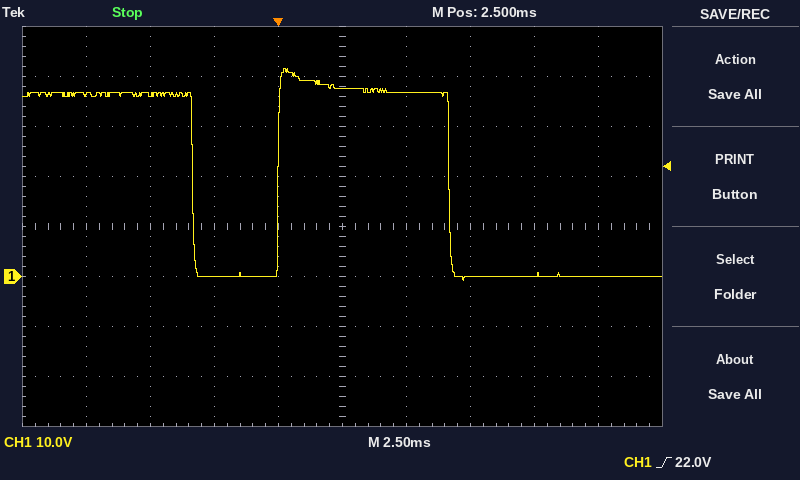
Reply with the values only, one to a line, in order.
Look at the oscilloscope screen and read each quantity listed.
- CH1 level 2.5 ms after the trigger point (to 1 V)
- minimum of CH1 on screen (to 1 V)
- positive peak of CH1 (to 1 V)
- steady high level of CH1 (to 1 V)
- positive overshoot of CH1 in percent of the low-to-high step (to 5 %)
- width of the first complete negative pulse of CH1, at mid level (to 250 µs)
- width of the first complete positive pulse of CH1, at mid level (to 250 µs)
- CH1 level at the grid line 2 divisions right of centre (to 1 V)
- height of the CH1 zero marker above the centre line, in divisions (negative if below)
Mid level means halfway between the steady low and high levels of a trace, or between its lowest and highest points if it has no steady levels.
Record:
38 V
-1 V
42 V
37 V
15 %
3.25 ms
6.75 ms
0 V
-1.0 div
